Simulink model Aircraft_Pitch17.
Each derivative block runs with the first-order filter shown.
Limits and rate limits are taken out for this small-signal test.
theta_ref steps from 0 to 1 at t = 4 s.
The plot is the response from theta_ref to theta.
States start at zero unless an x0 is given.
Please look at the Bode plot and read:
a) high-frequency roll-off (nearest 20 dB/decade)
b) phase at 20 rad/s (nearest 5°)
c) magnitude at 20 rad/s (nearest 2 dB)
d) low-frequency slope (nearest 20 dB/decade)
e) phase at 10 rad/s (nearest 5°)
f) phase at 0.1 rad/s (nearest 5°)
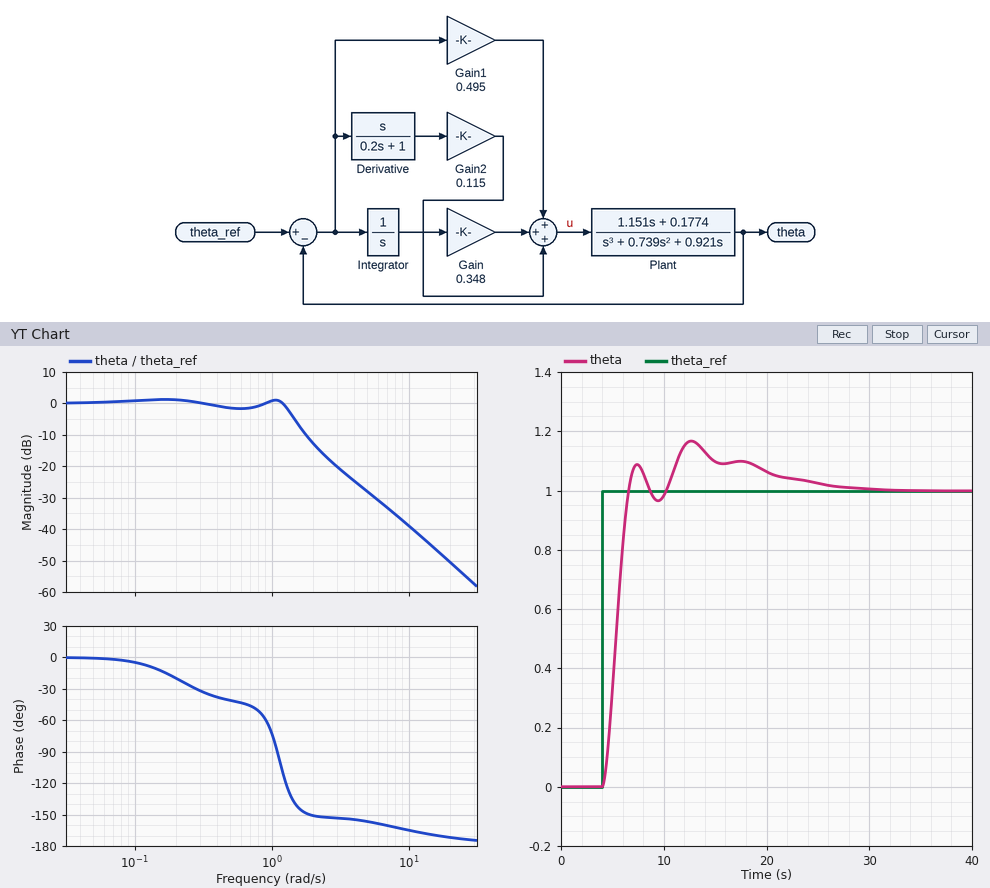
-40 dB/decade
-170°
-50 dB
0 dB/decade
-165°
-5°
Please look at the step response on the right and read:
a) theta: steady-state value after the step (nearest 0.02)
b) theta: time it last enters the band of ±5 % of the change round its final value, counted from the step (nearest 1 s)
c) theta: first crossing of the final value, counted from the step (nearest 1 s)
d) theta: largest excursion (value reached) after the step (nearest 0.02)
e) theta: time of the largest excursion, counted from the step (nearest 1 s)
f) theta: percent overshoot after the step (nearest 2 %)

1.00
17 s
3 s
1.16
9 s
16 %
